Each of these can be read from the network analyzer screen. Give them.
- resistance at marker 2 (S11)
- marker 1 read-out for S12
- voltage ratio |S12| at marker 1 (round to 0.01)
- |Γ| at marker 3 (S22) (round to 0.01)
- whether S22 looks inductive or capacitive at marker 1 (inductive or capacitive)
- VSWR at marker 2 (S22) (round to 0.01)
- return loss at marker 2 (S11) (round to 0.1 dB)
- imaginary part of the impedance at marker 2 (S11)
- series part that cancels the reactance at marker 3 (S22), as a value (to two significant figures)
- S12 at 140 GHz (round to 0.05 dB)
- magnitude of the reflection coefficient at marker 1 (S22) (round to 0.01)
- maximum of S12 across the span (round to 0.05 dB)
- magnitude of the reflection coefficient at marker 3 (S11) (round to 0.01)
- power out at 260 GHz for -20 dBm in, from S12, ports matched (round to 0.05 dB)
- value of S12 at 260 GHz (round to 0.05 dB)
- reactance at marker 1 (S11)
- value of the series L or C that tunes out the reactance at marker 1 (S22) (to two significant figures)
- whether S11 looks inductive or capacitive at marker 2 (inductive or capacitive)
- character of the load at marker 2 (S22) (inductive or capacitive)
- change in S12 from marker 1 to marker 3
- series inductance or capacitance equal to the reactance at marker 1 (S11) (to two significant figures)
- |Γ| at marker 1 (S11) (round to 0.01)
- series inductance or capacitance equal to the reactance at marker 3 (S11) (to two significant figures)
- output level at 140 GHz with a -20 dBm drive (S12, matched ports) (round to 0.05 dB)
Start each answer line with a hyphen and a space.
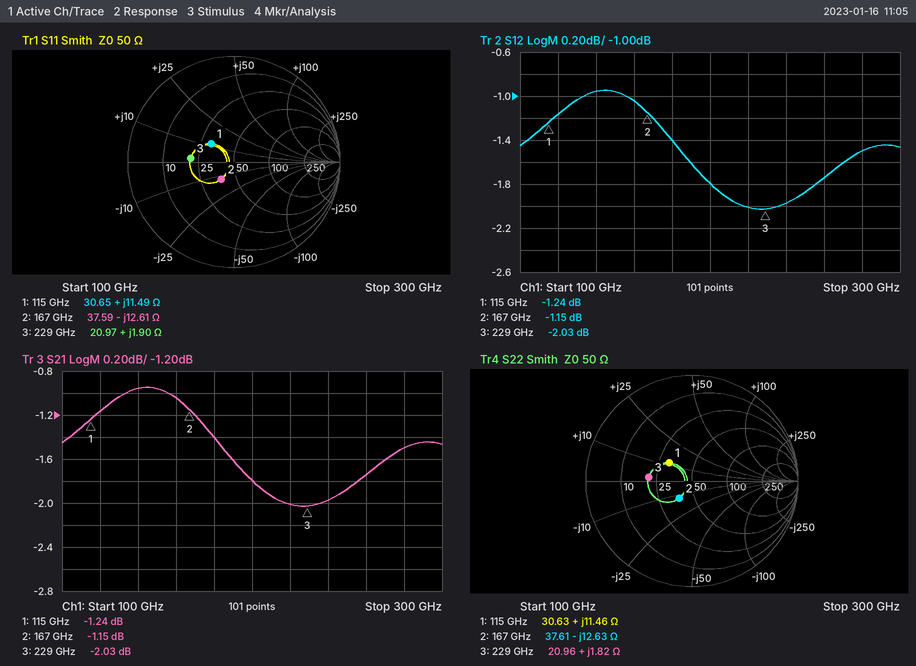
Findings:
- 37.59 Ω
- -1.24 dB
- 0.87
- 0.41
- inductive
- 1.50
- 14.0 dB
- -12.61 Ω
- 380 fF
- -0.95 dB
- 0.28
- -0.95 dB
- 0.41
- -21.75 dBm
- -1.75 dB
- +11.49 Ω
- 120 fF
- capacitive
- capacitive
- -0.79 dB
- 16 pH
- 0.28
- 1.3 pH
- -20.95 dBm
